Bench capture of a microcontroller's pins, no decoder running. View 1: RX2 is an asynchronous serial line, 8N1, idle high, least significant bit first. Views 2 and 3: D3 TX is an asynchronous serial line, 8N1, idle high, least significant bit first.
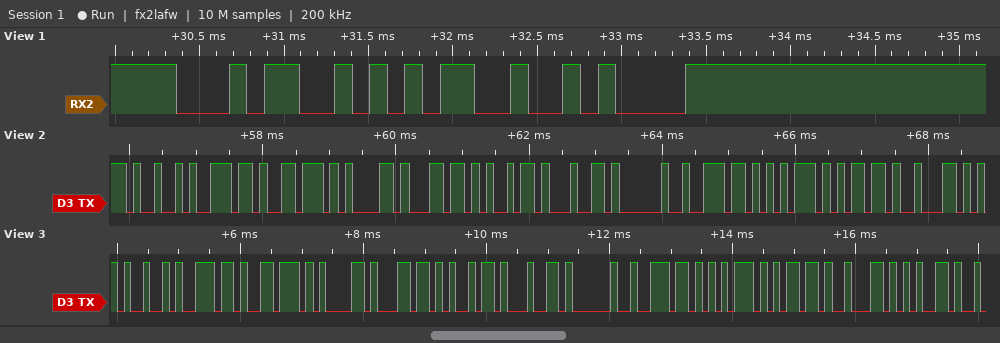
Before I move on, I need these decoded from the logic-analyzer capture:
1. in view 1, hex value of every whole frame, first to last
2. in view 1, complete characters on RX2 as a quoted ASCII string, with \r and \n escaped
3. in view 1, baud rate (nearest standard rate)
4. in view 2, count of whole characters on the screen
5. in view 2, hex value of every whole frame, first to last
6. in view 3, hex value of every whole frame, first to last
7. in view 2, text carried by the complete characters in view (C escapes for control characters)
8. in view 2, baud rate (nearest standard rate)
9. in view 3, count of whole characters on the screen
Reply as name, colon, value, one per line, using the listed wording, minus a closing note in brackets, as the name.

in view 1, hex value of every whole frame, first to last: 0x34 0x35 0x0A
in view 1, complete characters on RX2 as a quoted ASCII string, with \r and \n escaped: "45\n"
in view 1, baud rate: 9600 baud
in view 2, count of whole characters on the screen: 12
in view 2, hex value of every whole frame, first to last: 49 6E 76 61 6C 69 64 20 6E 75 6D 62
in view 3, hex value of every whole frame, first to last: 0x49 0x6E 0x76 0x61 0x6C 0x69 0x64 0x20 0x6E 0x75 0x6D 0x62 0x65
in view 2, text carried by the complete characters in view: "Invalid numb"
in view 2, baud rate: 9600 baud
in view 3, count of whole characters on the screen: 13
